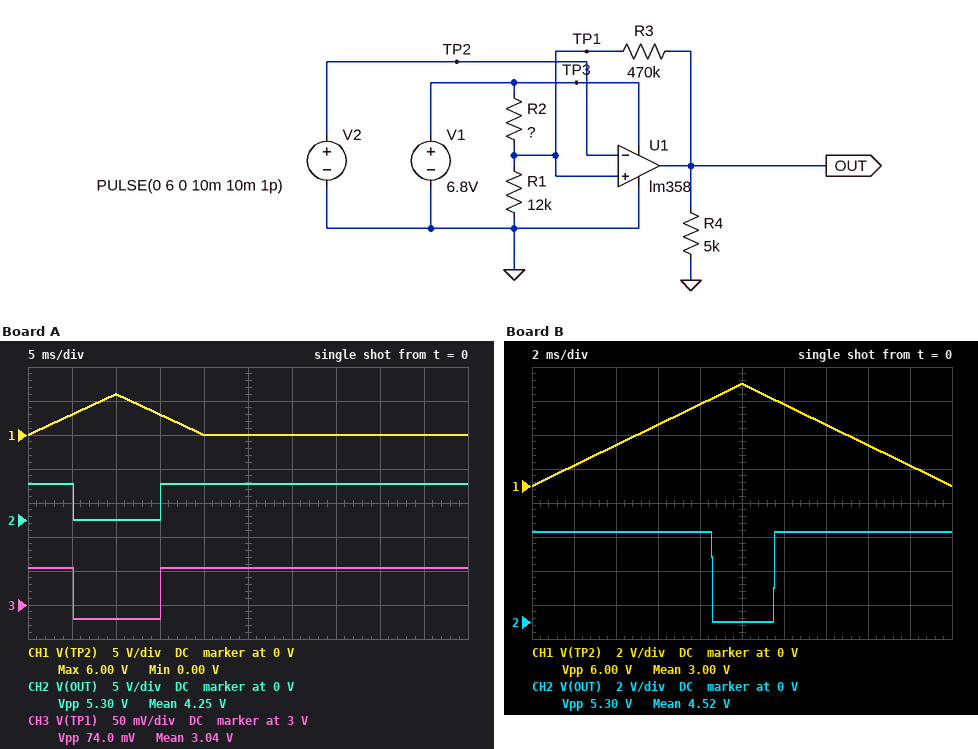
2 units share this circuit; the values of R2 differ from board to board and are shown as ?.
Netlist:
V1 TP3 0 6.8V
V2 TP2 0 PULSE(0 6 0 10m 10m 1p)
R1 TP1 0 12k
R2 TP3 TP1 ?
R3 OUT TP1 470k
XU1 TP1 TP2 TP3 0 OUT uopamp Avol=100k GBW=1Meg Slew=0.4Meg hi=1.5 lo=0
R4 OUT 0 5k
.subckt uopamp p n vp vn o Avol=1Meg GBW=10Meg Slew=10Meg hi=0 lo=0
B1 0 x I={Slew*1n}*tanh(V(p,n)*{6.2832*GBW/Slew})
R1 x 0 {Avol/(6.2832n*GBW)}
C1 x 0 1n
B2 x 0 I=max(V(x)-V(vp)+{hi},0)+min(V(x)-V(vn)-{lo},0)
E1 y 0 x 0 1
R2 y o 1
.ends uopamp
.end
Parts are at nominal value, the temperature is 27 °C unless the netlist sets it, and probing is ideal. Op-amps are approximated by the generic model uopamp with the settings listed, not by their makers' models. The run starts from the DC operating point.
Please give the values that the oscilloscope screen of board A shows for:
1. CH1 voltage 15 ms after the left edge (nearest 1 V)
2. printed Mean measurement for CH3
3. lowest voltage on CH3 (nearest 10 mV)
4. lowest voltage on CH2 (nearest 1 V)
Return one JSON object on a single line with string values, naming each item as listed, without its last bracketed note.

{"CH1 voltage 15 ms after the left edge": "3 V", "printed Mean measurement for CH3": "3.04 V", "lowest voltage on CH3": "2.98 V", "lowest voltage on CH2": "0 V"}
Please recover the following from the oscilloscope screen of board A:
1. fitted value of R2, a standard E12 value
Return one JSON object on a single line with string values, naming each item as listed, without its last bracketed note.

{"fitted value of R2, a standard E12 value": "15 kΩ"}
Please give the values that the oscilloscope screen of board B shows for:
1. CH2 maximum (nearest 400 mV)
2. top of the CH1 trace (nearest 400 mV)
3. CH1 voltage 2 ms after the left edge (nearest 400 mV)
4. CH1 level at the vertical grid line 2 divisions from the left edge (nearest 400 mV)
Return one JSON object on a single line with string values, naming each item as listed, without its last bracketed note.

{"CH2 maximum": "5.2 V", "top of the CH1 trace": "6.0 V", "CH1 voltage 2 ms after the left edge": "1.2 V", "CH1 level at the vertical grid line 2 divisions from the left edge": "2.4 V"}
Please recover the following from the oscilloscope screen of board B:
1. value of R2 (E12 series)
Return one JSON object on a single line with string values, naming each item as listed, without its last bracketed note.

{"value of R2": "3.9 kΩ"}
